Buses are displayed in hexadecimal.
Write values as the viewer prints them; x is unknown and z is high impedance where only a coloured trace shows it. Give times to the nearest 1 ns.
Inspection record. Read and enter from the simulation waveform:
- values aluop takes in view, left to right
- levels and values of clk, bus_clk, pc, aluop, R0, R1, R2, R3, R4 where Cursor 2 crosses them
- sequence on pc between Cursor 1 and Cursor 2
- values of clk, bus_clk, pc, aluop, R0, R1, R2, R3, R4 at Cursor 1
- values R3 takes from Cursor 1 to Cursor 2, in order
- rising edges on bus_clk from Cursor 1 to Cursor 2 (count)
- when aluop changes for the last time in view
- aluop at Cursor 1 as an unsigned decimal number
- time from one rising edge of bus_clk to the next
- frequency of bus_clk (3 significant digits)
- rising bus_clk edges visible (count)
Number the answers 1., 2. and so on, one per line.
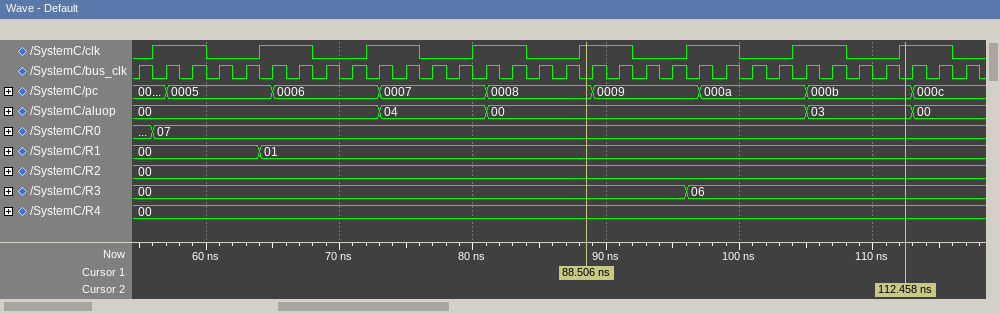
1. 00, 04, 00, 03, 00
2. clk=1, bus_clk=0, pc=000b, aluop=03, R0=07, R1=01, R2=00, R3=06, R4=00
3. 0008, 0009, 000a, 000b
4. clk=1, bus_clk=0, pc=0008, aluop=00, R0=07, R1=01, R2=00, R3=00, R4=00
5. 00, 06
6. 12
7. 113 ns
8. 0
9. 2 ns
10. 500 MHz
11. 32
